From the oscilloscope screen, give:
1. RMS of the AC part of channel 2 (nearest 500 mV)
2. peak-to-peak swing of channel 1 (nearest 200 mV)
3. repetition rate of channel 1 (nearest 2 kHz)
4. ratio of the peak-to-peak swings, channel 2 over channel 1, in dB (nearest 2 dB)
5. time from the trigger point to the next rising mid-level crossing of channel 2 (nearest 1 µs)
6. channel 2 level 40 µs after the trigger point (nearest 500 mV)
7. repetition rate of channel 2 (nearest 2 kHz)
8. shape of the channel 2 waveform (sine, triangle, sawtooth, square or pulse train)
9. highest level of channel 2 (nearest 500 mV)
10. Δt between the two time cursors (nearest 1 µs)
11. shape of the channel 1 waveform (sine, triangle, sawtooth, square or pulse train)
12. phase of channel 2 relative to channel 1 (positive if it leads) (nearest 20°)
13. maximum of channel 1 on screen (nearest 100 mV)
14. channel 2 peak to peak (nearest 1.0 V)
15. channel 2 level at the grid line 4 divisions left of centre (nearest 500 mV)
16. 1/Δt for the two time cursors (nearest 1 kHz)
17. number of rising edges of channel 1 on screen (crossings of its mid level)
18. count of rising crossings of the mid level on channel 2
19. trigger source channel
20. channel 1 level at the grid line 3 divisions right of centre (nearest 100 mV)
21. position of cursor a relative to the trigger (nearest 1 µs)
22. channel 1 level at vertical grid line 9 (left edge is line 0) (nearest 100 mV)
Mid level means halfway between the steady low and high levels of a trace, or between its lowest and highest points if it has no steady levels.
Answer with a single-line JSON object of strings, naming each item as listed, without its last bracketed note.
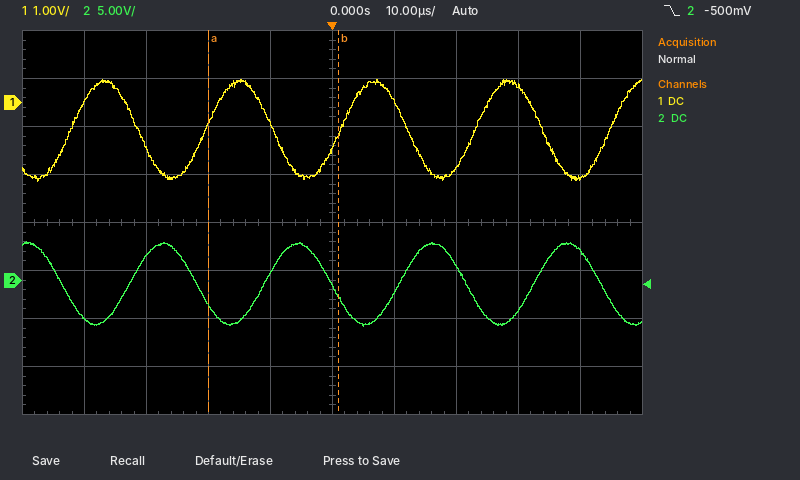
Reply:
{"RMS of the AC part of channel 2": "3.0 V", "peak-to-peak swing of channel 1": "2.2 V", "repetition rate of channel 1": "46 kHz", "ratio of the peak-to-peak swings, channel 2 over channel 1, in dB": "12 dB", "time from the trigger point to the next rising mid-level crossing of channel 2": "11 µs", "channel 2 level 40 µs after the trigger point": "3.0 V", "repetition rate of channel 2": "46 kHz", "shape of the channel 2 waveform": "sine", "highest level of channel 2": "4.0 V", "Δt between the two time cursors": "21 µs", "shape of the channel 1 waveform": "sine", "phase of channel 2 relative to channel 1 (positive if it leads)": "-160°", "maximum of channel 1 on screen": "500 mV", "channel 2 peak to peak": "9.0 V", "channel 2 level at the grid line 4 divisions left of centre": "-4.0 V", "1/Δt for the two time cursors": "48 kHz", "number of rising edges of channel 1 on screen": "5", "count of rising crossings of the mid level on channel 2": "4", "trigger source channel": "channel 2", "channel 1 level at the grid line 3 divisions right of centre": "300 mV", "position of cursor a relative to the trigger": "-20 µs", "channel 1 level at vertical grid line 9 (left edge is line 0)": "-1.6 V"}
